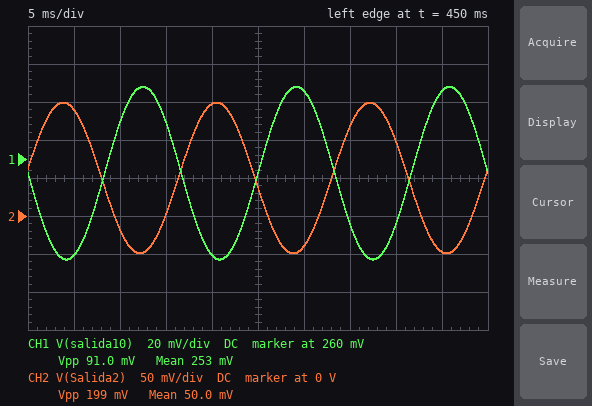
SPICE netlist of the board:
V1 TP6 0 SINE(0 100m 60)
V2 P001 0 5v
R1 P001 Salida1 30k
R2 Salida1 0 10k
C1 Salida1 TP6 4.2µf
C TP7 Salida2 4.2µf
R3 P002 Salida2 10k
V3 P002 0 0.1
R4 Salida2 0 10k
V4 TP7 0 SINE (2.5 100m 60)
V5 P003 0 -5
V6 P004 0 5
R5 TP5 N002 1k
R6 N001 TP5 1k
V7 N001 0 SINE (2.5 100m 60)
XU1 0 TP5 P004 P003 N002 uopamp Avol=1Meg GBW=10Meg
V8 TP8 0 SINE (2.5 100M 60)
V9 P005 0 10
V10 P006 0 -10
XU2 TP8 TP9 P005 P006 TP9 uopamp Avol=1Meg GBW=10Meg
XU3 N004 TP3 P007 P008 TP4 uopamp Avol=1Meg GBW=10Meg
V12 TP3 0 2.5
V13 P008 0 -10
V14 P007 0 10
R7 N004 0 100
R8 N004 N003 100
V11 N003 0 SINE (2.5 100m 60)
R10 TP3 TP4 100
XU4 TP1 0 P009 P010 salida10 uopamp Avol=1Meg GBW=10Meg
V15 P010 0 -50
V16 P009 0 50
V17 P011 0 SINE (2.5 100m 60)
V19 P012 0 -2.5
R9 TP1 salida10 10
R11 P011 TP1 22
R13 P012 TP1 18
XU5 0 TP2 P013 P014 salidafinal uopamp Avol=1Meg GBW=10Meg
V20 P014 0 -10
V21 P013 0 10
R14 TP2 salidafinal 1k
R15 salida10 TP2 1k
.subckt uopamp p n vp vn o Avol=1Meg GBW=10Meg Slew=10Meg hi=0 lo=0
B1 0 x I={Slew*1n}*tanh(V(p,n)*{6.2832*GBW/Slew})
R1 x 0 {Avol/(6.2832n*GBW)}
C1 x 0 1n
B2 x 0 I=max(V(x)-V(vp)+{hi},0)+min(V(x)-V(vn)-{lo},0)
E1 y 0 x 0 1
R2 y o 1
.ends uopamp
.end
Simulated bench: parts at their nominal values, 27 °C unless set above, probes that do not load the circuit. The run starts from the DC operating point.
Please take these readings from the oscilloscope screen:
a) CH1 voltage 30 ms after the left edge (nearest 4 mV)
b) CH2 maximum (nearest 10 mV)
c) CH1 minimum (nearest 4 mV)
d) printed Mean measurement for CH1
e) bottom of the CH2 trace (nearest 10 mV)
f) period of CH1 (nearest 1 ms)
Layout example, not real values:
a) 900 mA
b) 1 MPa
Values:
a) 296 mV
b) 150 mV
c) 208 mV
d) 253 mV
e) -50 mV
f) 17 ms
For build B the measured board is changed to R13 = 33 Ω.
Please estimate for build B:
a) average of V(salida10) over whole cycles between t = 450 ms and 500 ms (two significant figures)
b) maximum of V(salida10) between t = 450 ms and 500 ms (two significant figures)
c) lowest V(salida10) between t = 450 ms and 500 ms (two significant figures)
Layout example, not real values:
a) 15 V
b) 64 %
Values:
a) -380 mV
b) -330 mV
c) -420 mV
